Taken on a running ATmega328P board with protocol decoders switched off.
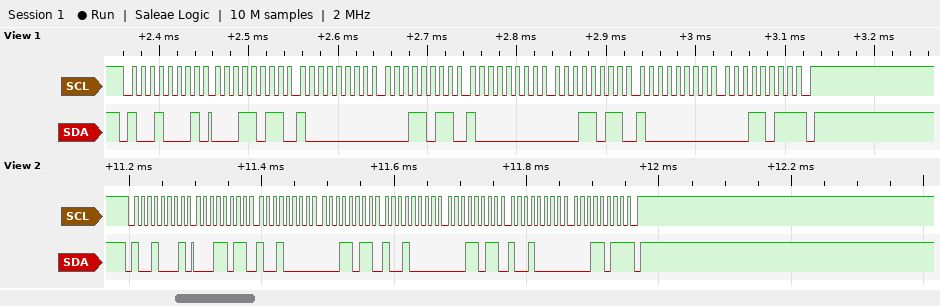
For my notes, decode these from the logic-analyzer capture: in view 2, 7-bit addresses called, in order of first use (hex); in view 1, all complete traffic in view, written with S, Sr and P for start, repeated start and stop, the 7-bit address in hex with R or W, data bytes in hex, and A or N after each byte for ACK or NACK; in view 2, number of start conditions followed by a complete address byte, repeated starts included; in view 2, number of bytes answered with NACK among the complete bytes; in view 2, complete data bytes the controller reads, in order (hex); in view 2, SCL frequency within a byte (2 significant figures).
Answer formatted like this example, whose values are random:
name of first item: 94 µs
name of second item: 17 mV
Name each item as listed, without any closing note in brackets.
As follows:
in view 2, 7-bit addresses called, in order of first use: 0x48
in view 1, all complete traffic in view, written with S, Sr and P for start, repeated start and stop, the 7-bit address in hex with R or W, data bytes in hex, and A or N after each byte for ACK or NACK: S 48R A 1B A 80 A 1B A 80 A 1B A 80 A 1B N P
in view 2, number of start conditions followed by a complete address byte, repeated starts included: 1
in view 2, number of bytes answered with NACK among the complete bytes: 1
in view 2, complete data bytes the controller reads, in order: 1B 90 1B 90 1B 90 1B
in view 2, SCL frequency within a byte: 100 kHz
